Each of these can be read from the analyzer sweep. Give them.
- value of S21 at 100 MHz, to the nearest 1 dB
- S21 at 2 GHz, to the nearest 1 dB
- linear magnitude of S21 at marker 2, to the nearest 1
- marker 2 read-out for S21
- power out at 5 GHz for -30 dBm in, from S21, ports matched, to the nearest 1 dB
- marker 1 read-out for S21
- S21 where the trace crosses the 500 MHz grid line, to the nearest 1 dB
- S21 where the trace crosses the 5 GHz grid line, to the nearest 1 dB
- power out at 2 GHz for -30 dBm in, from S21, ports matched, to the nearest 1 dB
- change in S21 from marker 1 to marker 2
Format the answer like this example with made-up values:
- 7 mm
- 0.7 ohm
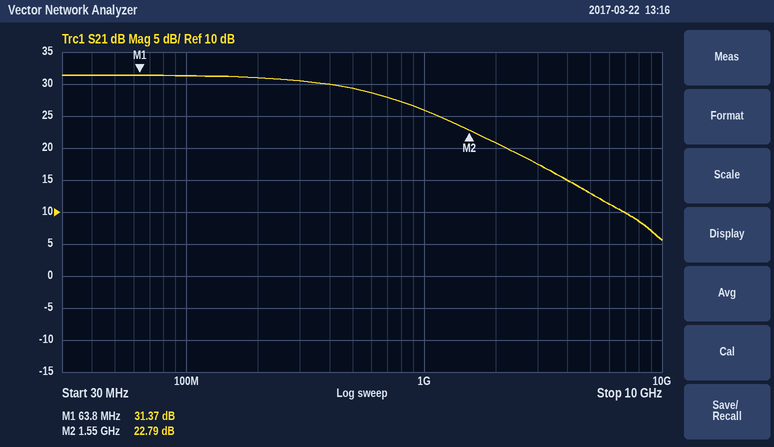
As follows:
- 31 dB
- 21 dB
- 14
- 22.79 dB
- -17 dBm
- 31.37 dB
- 29 dB
- 13 dB
- -9 dBm
- -8.58 dB
